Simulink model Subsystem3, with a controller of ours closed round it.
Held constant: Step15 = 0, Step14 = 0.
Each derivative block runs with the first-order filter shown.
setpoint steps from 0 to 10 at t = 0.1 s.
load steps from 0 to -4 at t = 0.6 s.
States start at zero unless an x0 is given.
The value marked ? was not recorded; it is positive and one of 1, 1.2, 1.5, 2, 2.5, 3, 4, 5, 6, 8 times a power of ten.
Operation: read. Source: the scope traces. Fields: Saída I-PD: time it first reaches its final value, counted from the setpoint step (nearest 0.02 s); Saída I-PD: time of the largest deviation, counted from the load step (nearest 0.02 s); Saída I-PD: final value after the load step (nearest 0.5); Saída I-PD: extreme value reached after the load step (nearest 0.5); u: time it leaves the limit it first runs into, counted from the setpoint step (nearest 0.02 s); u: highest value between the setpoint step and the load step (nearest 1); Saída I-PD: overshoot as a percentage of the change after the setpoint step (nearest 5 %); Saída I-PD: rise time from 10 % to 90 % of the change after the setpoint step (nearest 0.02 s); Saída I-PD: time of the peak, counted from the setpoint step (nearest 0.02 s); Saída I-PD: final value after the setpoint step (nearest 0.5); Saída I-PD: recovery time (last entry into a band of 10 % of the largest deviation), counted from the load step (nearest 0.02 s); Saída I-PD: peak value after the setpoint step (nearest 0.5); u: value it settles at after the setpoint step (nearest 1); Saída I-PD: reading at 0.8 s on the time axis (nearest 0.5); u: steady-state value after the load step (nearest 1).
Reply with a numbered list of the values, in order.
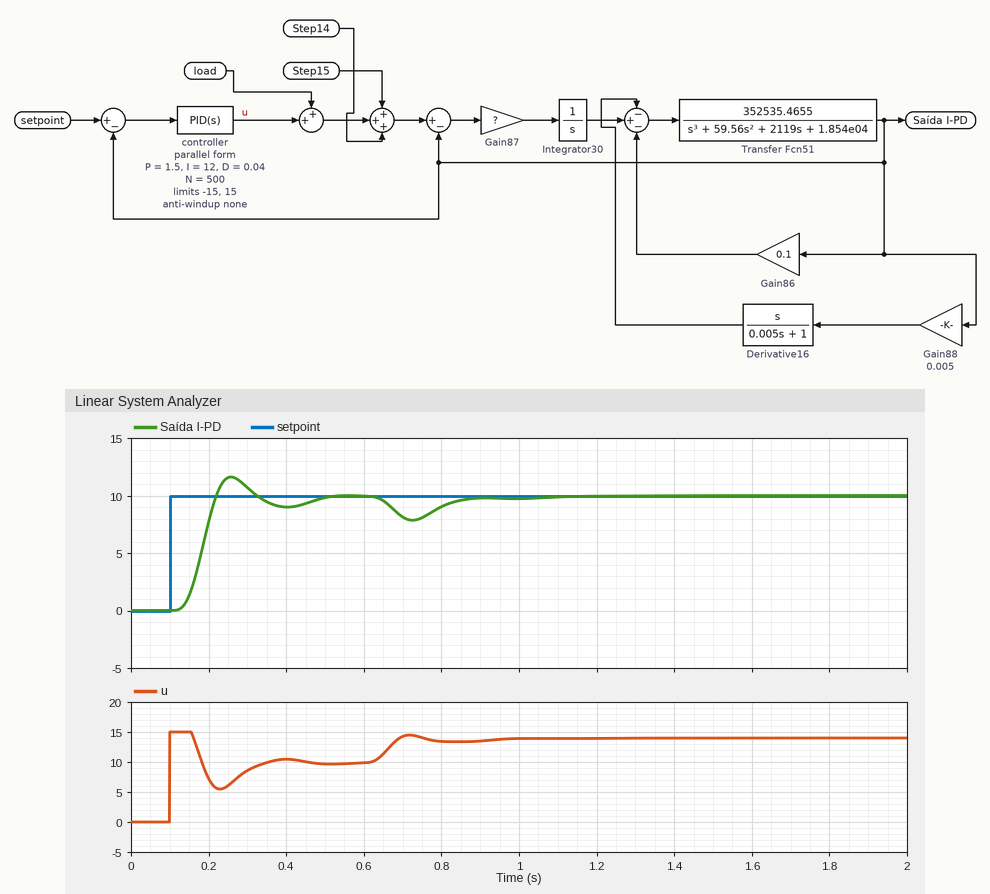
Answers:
1. 0.12 s
2. 0.12 s
3. 10.0
4. 8.0
5. 0.06 s
6. 15
7. 15 %
8. 0.06 s
9. 0.16 s
10. 10.0
11. 0.46 s
12. 11.5
13. 10
14. 9.0
15. 14
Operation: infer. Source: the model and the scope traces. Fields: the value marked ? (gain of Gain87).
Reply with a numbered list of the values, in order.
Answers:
1. 2
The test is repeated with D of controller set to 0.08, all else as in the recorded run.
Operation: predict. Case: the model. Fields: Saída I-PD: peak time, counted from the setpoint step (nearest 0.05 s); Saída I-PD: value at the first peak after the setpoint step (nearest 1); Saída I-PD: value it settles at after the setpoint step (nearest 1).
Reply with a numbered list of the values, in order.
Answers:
1. 0.25 s
2. 11
3. 10
